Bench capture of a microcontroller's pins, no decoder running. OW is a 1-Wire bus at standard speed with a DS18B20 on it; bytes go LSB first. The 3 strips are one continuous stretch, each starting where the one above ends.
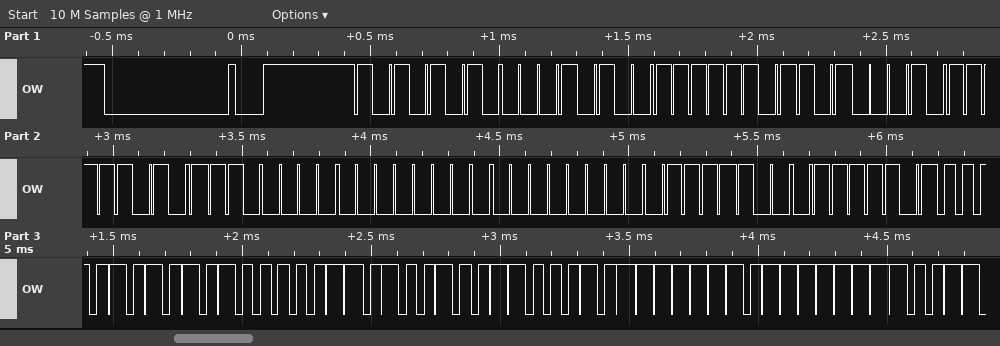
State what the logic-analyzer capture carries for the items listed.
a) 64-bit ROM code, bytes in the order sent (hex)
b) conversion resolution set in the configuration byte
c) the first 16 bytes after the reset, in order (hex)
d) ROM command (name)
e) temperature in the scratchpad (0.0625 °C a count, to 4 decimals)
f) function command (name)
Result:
28 BF 45 5F 07 00 00 3E
12 bits
55 28 BF 45 5F 07 00 00 3E BE 50 05 4B 46 7F FF
Match ROM
85.0000 °C
Read Scratchpad
